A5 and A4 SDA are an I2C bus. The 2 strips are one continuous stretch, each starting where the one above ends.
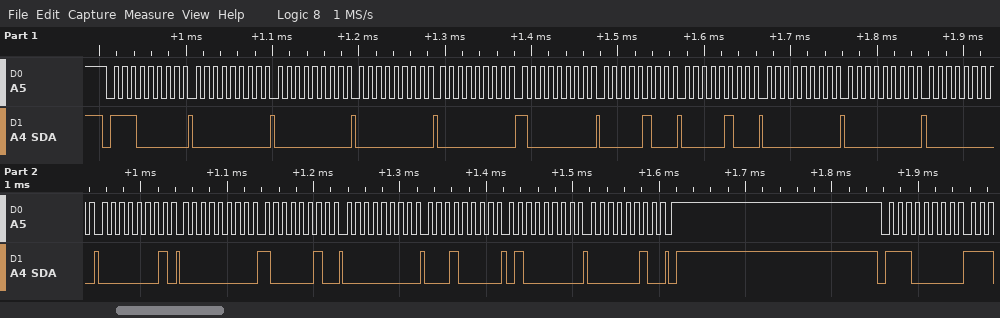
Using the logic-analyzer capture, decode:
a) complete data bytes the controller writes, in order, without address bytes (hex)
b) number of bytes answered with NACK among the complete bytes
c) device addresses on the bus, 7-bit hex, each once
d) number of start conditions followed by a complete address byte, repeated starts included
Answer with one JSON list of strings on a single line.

["00 00 00 00 80 04 04 00 00 00 01 00 82 00 10 40 02", "0", "0x70", "2"]
